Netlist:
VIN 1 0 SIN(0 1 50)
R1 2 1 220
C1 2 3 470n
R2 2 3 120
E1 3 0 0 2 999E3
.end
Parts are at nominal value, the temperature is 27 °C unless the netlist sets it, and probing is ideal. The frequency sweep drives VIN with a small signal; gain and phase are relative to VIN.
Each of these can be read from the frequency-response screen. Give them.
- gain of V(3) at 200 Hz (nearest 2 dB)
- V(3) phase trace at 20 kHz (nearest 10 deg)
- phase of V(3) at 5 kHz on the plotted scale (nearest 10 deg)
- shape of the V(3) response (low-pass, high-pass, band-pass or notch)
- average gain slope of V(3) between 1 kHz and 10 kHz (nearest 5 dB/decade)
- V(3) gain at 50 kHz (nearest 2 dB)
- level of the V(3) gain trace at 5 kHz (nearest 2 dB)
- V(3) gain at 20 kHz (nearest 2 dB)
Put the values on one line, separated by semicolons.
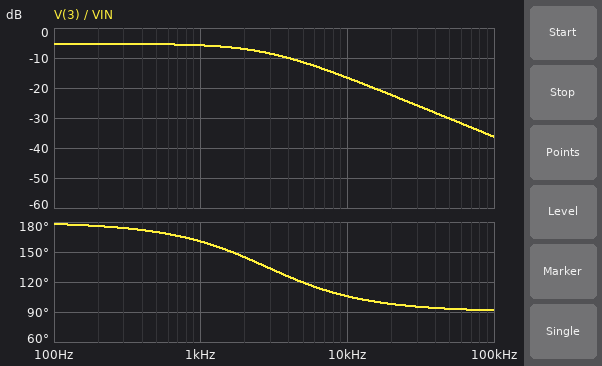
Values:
-6 dB; 100 deg; 120 deg; low-pass; -10 dB/decade; -30 dB; -12 dB; -22 dB
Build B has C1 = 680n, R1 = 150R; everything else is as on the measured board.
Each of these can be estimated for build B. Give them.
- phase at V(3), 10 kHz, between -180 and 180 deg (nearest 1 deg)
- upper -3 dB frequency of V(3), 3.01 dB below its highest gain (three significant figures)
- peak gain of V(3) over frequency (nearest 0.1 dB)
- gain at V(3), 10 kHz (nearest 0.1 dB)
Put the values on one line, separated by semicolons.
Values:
101 deg; 1.95 kHz; -1.9 dB; -16.3 dB
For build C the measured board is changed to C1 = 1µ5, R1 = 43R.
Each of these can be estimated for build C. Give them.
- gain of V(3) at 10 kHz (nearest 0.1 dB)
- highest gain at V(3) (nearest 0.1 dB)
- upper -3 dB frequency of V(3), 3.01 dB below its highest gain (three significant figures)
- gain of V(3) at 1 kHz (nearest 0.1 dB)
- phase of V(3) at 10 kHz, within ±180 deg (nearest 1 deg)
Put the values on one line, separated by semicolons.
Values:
-12.2 dB; 8.9 dB; 884 Hz; 5.3 dB; 95 deg
